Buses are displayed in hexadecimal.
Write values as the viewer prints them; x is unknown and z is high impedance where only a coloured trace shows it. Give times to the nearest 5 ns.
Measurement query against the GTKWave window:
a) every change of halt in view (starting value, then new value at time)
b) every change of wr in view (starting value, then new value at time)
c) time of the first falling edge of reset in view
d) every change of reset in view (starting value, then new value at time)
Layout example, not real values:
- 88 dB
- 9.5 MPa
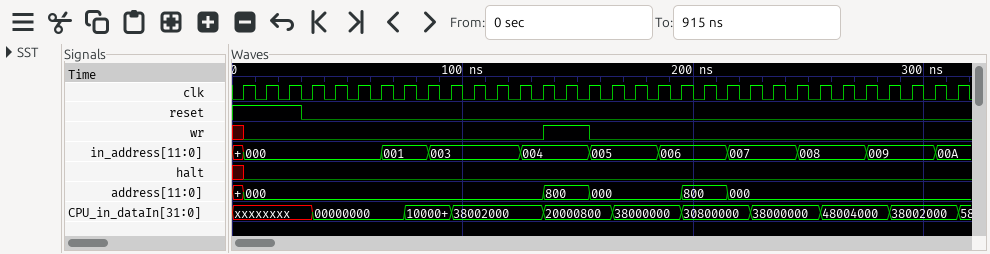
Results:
- x, 0 at 5 ns
- x, 0 at 5 ns, 1 at 135 ns, 0 at 155 ns
- 30 ns
- 1, 0 at 30 ns
